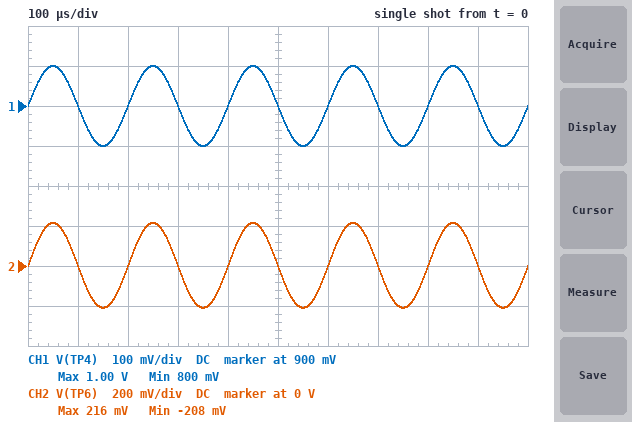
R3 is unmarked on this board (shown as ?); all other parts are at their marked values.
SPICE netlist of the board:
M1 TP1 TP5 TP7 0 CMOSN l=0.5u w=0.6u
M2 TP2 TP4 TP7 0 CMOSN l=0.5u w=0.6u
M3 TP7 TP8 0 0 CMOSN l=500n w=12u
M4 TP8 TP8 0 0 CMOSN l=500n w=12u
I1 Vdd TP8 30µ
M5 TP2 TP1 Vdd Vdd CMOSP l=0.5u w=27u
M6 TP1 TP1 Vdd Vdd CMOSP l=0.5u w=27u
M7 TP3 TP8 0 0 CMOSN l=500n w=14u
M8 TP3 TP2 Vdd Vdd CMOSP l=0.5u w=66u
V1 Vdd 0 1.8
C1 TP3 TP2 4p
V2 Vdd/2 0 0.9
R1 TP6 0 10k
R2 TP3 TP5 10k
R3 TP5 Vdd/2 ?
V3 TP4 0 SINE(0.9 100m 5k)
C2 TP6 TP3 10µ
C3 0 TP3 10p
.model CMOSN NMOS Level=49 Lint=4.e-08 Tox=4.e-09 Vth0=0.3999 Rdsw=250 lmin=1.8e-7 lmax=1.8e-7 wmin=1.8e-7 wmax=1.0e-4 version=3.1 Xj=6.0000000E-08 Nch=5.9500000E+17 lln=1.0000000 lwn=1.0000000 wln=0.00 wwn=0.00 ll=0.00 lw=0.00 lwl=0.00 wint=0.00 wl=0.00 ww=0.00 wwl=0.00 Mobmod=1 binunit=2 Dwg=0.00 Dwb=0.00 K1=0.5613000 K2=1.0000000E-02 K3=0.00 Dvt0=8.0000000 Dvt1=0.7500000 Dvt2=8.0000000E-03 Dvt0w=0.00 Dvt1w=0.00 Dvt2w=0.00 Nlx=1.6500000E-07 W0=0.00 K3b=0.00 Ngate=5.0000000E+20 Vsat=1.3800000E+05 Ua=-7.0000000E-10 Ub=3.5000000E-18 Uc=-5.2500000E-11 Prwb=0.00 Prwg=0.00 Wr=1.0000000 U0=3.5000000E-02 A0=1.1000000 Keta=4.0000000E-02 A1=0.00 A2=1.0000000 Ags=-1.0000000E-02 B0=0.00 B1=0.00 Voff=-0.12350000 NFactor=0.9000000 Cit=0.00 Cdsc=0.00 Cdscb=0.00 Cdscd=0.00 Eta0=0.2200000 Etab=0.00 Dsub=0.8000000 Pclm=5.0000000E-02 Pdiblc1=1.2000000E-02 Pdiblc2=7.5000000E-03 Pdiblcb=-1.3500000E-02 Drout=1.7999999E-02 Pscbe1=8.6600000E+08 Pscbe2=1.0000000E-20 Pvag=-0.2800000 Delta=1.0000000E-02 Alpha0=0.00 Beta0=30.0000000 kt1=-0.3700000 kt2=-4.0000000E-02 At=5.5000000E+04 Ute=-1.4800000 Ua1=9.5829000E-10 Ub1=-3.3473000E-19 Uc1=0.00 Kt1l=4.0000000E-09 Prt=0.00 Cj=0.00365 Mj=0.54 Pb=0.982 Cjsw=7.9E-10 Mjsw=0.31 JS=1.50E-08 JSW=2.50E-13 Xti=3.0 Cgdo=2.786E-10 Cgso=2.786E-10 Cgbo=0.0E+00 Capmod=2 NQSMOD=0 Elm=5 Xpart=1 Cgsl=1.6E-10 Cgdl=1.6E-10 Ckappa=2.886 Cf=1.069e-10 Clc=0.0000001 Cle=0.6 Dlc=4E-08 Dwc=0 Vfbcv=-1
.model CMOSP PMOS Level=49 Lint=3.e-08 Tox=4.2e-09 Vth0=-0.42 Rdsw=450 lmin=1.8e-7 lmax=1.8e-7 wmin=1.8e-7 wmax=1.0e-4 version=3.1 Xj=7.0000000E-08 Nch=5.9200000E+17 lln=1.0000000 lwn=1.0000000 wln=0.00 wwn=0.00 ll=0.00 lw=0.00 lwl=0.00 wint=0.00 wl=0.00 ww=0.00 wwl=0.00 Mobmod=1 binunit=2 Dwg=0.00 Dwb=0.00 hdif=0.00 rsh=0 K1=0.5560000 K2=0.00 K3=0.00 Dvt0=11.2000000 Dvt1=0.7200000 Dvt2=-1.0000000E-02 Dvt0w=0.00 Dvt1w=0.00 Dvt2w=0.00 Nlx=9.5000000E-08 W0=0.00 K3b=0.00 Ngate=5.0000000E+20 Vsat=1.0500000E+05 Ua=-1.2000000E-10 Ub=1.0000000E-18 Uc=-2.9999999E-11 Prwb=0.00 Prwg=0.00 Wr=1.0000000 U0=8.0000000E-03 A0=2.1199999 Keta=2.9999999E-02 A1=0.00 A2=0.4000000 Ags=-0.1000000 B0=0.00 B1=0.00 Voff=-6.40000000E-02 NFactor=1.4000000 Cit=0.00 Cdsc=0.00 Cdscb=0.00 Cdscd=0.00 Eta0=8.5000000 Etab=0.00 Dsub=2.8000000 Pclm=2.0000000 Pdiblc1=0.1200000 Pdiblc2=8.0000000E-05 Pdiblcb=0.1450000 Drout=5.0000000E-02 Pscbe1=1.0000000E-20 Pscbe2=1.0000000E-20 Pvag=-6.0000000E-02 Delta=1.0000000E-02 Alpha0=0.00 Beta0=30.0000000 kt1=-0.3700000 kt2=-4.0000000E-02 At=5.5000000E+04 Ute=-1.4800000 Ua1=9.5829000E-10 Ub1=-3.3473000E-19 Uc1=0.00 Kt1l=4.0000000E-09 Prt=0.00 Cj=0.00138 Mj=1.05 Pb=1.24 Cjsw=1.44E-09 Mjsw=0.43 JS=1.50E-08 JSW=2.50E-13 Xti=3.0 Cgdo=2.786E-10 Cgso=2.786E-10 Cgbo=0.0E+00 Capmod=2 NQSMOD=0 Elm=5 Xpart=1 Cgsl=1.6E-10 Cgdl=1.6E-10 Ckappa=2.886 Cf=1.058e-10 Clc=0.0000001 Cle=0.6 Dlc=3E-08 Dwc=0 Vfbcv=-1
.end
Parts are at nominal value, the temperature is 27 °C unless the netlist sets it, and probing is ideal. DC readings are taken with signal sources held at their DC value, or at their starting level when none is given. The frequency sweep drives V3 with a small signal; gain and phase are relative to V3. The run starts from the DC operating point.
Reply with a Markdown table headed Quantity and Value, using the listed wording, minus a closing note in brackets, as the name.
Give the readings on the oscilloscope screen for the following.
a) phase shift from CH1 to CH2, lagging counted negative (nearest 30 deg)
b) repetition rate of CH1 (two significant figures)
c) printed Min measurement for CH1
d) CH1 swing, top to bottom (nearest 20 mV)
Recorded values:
| Quantity | Value |
|---|---|
| phase shift from CH1 to CH2, lagging counted negative | 0 deg |
| repetition rate of CH1 | 5.0 kHz |
| printed Min measurement for CH1 | 800 mV |
| CH1 swing, top to bottom | 200 mV |
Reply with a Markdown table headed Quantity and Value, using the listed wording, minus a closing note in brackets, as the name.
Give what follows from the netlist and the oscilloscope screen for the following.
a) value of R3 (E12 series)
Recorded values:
| Quantity | Value |
|---|---|
| value of R3 | 8.2 kΩ |
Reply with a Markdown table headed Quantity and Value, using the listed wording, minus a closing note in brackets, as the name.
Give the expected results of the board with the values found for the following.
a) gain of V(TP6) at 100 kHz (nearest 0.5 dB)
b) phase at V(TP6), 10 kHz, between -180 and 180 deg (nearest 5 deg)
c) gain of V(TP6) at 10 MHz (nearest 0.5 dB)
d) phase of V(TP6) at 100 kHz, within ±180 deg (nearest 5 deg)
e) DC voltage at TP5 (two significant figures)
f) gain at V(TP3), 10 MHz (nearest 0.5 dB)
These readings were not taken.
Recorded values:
| Quantity | Value |
|---|---|
| gain of V(TP6) at 100 kHz | 6.5 dB |
| phase at V(TP6), 10 kHz, between -180 and 180 deg | 0 deg |
| gain of V(TP6) at 10 MHz | -13.5 dB |
| phase of V(TP6) at 100 kHz, within ±180 deg | -5 deg |
| DC voltage at TP5 | 900 mV |
| gain at V(TP3), 10 MHz | -13.5 dB |
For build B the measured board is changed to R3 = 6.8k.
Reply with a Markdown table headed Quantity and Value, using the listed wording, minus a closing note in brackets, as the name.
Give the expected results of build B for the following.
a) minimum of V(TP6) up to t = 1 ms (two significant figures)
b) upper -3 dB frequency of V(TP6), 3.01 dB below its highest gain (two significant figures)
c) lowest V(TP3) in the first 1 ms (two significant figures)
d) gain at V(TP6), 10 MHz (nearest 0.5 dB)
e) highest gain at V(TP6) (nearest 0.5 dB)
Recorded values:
| Quantity | Value |
|---|---|
| minimum of V(TP6) up to t = 1 ms | -220 mV |
| upper -3 dB frequency of V(TP6), 3.01 dB below its highest gain | 1.1 MHz |
| lowest V(TP3) in the first 1 ms | 680 mV |
| gain at V(TP6), 10 MHz | -14.0 dB |
| highest gain at V(TP6) | 7.5 dB |
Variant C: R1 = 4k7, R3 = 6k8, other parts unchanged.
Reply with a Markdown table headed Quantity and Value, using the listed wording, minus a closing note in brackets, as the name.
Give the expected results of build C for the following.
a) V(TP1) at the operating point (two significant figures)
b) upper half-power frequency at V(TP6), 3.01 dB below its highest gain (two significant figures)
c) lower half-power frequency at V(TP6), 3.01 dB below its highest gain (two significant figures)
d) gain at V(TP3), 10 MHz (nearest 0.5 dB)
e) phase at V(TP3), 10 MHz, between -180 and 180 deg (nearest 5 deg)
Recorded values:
| Quantity | Value |
|---|---|
| V(TP1) at the operating point | 1.2 V |
| upper half-power frequency at V(TP6), 3.01 dB below its highest gain | 970 kHz |
| lower half-power frequency at V(TP6), 3.01 dB below its highest gain | 3.2 Hz |
| gain at V(TP3), 10 MHz | -14.5 dB |
| phase at V(TP3), 10 MHz, between -180 and 180 deg | -145 deg |
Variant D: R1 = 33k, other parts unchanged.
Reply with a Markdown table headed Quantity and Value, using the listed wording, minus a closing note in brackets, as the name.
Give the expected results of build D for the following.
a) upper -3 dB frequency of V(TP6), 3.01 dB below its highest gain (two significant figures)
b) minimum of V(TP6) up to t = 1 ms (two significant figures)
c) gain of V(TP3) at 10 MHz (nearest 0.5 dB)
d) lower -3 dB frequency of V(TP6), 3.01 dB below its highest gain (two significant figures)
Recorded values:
| Quantity | Value |
|---|---|
| upper -3 dB frequency of V(TP6), 3.01 dB below its highest gain | 1.4 MHz |
| minimum of V(TP6) up to t = 1 ms | -220 mV |
| gain of V(TP3) at 10 MHz | -13.0 dB |
| lower -3 dB frequency of V(TP6), 3.01 dB below its highest gain | 480 mHz |
